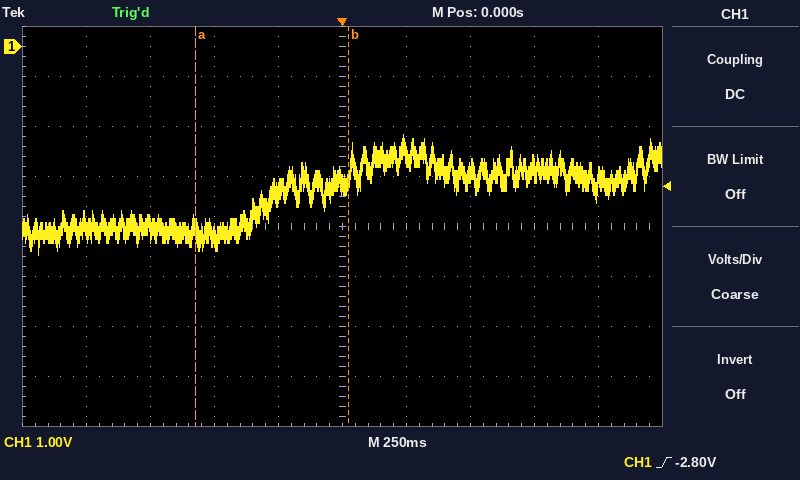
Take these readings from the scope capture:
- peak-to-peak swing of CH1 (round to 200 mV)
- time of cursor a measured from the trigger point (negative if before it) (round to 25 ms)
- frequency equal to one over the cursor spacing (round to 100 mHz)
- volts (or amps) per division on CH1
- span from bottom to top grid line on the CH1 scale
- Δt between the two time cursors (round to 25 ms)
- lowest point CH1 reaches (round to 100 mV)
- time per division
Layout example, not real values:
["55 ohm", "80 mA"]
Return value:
["2.4 V", "-575 ms", "1.7 Hz", "1 V", "8 V", "600 ms", "-4.2 V", "250 ms"]
